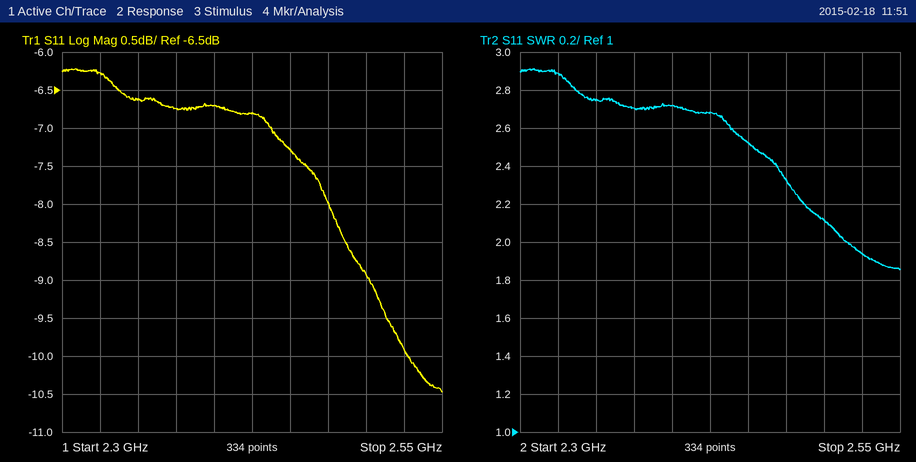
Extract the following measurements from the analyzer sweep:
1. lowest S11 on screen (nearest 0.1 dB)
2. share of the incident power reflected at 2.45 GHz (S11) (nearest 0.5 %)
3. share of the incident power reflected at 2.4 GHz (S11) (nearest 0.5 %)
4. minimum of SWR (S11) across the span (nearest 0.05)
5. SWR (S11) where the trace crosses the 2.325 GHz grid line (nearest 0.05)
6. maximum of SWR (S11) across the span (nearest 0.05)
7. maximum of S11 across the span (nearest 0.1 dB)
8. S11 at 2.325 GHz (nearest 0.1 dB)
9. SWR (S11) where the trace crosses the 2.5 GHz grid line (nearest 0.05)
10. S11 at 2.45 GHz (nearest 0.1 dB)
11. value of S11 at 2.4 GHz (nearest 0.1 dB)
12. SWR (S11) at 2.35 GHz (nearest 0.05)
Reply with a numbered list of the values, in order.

1. -10.5 dB
2. 18.5 %
3. 21.5 %
4. 1.85
5. 2.90
6. 2.90
7. -6.2 dB
8. -6.3 dB
9. 2.10
10. -7.3 dB
11. -6.7 dB
12. 2.75
